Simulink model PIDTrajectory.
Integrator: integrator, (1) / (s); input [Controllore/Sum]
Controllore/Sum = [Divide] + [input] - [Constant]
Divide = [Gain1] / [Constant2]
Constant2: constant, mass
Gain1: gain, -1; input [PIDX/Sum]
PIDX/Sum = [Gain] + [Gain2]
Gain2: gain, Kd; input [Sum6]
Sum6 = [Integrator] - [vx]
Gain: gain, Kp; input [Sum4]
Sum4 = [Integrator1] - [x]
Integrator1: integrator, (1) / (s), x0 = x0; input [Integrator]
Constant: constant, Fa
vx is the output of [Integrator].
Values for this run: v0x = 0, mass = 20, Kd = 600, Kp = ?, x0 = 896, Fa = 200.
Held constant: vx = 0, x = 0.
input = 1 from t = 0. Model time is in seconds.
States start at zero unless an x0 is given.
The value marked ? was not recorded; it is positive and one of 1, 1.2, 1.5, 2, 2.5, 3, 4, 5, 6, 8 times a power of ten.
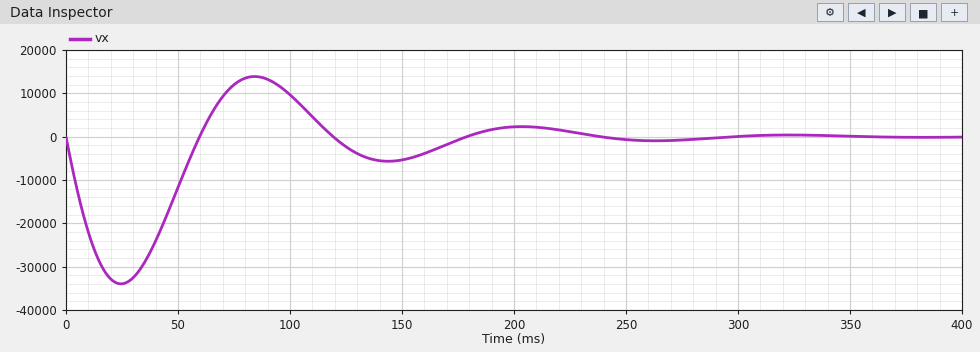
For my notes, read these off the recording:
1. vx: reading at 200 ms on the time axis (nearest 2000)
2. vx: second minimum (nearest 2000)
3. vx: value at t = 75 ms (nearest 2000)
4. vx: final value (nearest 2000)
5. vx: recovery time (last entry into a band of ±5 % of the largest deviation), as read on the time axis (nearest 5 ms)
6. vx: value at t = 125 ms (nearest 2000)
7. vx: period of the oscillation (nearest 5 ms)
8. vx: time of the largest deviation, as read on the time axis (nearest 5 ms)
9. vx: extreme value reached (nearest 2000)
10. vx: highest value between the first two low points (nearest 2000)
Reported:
2000
-6000
12000
0
220 ms
-2000
120 ms
25 ms
-34000
14000
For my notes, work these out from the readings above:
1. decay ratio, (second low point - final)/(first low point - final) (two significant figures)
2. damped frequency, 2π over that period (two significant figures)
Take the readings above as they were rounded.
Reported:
0.18
0.052 rad/ms
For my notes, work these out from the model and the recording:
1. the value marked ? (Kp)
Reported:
60000
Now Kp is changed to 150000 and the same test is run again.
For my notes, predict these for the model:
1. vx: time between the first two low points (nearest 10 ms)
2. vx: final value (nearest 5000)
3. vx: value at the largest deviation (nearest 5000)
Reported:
70 ms
0
-60000
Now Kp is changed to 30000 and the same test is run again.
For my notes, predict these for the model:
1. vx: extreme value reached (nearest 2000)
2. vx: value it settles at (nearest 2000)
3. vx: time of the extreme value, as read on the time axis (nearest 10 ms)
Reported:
-22000
0
30 ms
